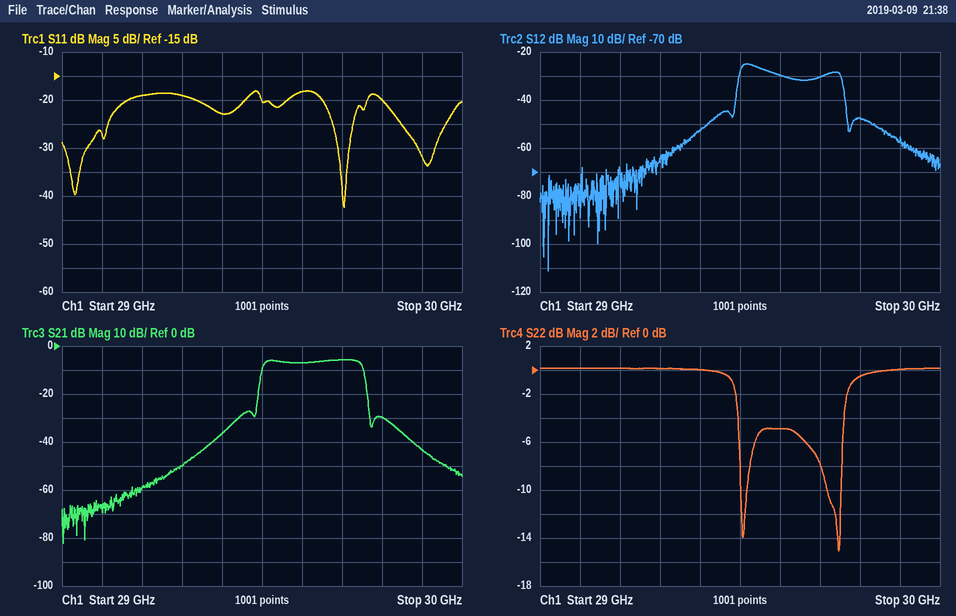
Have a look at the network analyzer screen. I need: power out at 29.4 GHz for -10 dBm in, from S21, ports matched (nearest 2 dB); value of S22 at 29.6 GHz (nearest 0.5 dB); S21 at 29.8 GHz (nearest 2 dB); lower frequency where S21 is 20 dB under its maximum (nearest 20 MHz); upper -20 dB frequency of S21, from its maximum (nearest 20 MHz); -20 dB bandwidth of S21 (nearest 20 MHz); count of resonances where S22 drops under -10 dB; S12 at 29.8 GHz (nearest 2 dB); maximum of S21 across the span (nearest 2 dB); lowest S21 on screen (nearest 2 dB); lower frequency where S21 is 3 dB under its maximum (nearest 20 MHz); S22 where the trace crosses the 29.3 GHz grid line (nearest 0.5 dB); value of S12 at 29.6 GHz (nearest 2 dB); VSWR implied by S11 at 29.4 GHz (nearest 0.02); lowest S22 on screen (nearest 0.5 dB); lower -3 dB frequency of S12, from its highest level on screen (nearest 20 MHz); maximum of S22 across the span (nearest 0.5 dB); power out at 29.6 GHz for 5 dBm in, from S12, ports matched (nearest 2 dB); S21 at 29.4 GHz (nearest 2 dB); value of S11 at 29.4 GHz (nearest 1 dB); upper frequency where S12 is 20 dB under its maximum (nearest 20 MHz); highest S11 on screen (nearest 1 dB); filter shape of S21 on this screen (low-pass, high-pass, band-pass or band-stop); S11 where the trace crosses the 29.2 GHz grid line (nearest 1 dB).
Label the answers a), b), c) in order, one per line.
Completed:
a) -46 dBm
b) -5.0 dB
c) -30 dB
d) 29.48 GHz
e) 29.76 GHz
f) 280 MHz
g) 2
h) -48 dB
i) -6 dB
j) -82 dB
k) 29.50 GHz
l) 0.0 dB
m) -30 dB
n) 1.16
o) -15.0 dB
p) 29.50 GHz
q) 0.0 dB
r) -24 dBm
s) -36 dB
t) -23 dB
u) 29.76 GHz
v) -18 dB
w) band-pass
x) -19 dB
